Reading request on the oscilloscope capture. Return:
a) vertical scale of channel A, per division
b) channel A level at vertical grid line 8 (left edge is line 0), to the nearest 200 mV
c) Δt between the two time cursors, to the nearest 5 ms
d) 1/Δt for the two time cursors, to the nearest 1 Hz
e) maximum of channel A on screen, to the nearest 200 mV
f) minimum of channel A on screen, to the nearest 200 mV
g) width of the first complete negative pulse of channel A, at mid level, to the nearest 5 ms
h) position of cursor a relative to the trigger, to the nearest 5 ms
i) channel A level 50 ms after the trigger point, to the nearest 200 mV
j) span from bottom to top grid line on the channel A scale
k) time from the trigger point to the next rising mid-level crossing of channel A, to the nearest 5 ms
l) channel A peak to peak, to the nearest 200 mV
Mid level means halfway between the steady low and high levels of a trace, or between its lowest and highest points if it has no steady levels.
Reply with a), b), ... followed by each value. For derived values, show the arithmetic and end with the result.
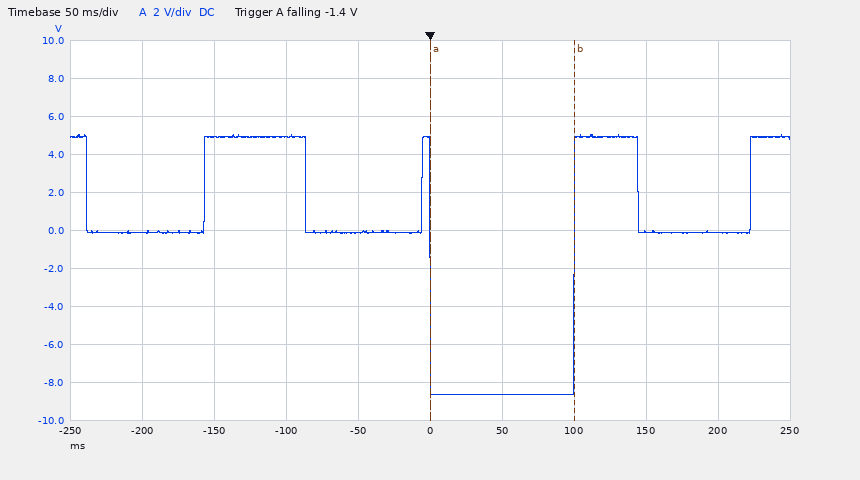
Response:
a) 2 V
b) 0.0 V
c) 100 ms
d) 1 / 100 ms ≈ 10 Hz
e) 5.0 V
f) -8.6 V
g) 100 ms
h) 0 ms
i) -8.6 V
j) 20 V
k) 100 ms
l) 5.0 V − (-8.6 V) = 13.6 V
